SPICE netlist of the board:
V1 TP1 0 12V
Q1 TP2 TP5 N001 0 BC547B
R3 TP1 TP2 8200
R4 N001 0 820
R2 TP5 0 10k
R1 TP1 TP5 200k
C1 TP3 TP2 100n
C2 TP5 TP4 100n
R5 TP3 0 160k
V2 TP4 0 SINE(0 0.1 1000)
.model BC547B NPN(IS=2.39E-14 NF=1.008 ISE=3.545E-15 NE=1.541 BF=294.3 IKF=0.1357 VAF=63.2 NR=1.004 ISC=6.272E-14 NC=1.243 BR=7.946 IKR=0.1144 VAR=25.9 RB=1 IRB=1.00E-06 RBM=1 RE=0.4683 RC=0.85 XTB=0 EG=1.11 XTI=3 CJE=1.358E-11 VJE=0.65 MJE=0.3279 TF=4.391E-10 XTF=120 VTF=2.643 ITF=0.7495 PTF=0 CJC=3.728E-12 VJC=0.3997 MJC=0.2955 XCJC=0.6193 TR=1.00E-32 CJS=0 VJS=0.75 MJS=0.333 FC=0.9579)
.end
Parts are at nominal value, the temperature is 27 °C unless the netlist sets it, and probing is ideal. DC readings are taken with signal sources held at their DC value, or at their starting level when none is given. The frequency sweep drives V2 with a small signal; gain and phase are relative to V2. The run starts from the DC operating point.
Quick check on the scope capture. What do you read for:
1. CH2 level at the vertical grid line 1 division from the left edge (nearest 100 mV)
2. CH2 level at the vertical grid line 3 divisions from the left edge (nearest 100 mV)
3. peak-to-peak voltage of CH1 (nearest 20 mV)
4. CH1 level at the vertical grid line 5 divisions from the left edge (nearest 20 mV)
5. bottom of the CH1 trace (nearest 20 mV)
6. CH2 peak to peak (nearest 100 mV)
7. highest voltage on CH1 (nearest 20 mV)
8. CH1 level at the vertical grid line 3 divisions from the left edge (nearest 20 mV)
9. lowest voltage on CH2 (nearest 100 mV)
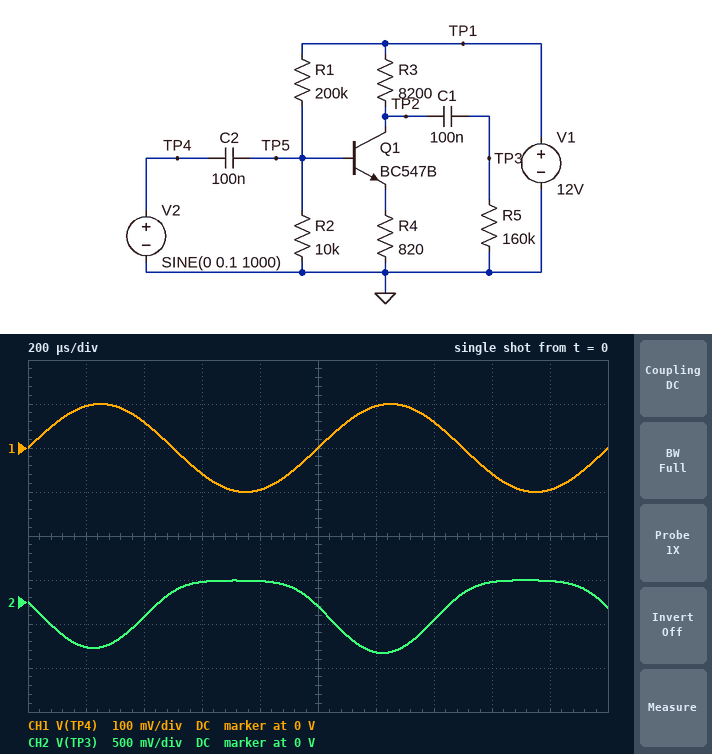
-500 mV
200 mV
200 mV
0 V
-100 mV
800 mV
100 mV
-60 mV
-600 mV
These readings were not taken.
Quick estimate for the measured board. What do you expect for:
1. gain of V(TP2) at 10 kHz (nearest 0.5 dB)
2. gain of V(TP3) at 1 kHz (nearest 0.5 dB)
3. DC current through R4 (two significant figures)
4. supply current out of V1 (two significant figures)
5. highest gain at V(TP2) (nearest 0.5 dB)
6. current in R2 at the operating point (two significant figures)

13.5 dB
13.5 dB
32 µA
89 µA
13.5 dB
57 µA
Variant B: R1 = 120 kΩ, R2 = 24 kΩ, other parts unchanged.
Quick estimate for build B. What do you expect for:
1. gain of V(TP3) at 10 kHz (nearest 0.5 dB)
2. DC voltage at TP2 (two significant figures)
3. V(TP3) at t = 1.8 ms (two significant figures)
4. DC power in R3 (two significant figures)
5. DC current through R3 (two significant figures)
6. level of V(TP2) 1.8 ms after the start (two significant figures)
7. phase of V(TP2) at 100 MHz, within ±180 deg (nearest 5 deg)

5.0 dB
1.2 V
1.0 V
14 mW
1.3 mA
2.2 V
0 deg
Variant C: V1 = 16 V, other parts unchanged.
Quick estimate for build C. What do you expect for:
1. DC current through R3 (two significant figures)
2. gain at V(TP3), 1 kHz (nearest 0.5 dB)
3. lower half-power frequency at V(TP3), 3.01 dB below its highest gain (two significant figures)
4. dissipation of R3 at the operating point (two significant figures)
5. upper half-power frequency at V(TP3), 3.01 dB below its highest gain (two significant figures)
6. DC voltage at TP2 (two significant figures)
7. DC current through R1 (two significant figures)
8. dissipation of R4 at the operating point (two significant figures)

200 µA
18.0 dB
170 Hz
330 µW
15 MHz
14 V
76 µA
33 µW
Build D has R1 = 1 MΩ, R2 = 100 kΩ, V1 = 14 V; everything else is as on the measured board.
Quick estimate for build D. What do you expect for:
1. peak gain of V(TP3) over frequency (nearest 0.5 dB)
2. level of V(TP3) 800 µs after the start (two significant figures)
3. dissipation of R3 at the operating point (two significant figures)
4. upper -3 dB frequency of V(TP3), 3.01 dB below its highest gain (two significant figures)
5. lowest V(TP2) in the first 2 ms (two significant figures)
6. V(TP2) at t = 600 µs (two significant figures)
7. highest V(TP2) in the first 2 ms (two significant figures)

19.0 dB
860 mV
2.8 mW
14 MHz
8.3 V
9.7 V
10 V
